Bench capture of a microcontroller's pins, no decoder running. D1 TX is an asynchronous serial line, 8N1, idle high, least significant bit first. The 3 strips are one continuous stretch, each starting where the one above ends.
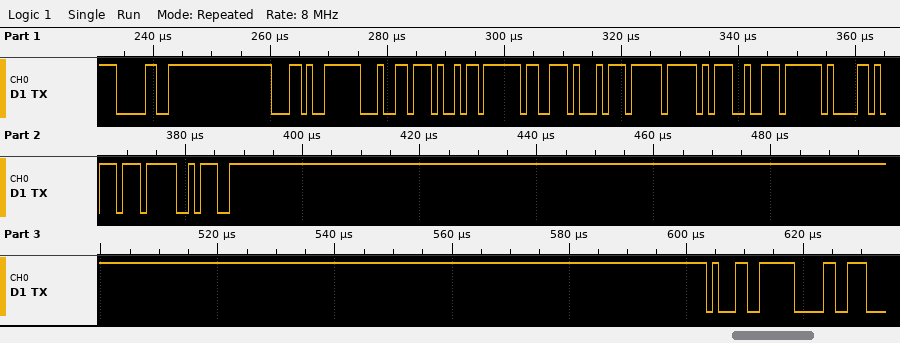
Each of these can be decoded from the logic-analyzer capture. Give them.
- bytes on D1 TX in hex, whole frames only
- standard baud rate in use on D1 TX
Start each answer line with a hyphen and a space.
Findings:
- 0x30 0x2C 0x64 0x69 0x73 0x74 0x5F 0x72 0x61 0x77 0x3A 0x31 0x30
- 1000000 baud
